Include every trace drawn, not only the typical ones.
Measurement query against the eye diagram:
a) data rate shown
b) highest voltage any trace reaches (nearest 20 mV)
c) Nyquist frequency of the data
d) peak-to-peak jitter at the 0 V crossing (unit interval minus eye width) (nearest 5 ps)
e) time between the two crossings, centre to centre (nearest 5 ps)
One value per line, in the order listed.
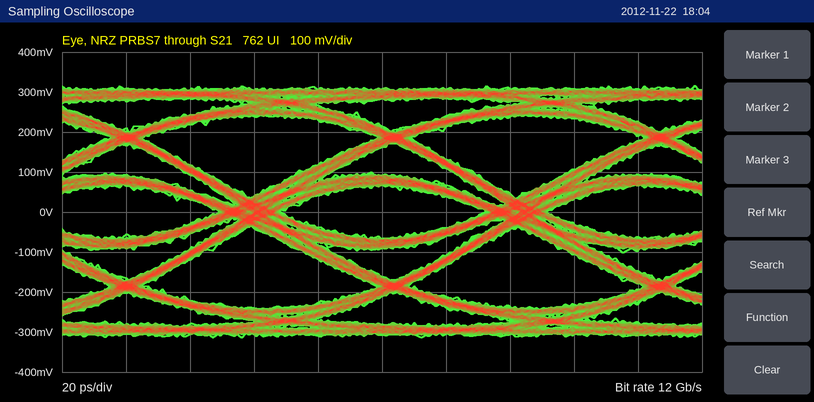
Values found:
12 Gb/s
320 mV
6 GHz
20 ps
85 ps
